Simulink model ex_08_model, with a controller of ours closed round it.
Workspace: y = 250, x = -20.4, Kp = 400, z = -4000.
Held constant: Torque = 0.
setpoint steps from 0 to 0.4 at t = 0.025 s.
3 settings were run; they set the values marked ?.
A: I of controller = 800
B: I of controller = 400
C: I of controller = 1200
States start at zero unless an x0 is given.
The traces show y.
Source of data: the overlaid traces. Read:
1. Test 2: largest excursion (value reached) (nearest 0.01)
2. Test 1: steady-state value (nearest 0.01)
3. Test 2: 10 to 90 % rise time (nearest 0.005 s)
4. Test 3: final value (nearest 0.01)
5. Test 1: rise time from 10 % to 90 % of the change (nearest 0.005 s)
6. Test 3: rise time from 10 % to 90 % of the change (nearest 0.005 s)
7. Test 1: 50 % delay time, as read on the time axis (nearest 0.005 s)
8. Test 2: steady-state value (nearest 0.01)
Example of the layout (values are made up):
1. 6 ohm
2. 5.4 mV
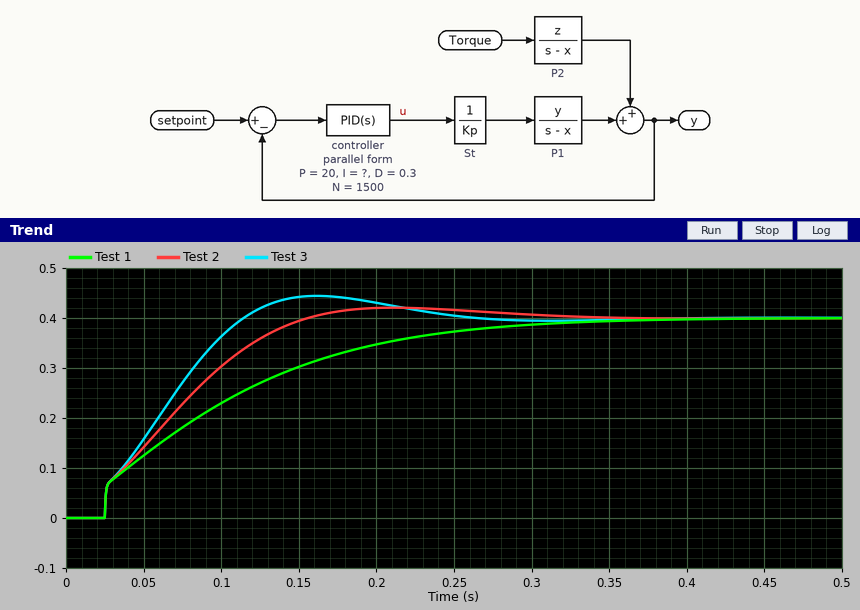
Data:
1. 0.42
2. 0.40
3. 0.100 s
4. 0.40
5. 0.195 s
6. 0.075 s
7. 0.085 s
8. 0.40
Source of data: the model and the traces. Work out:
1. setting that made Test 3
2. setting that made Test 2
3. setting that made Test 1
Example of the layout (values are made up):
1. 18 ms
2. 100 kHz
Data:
1. C
2. A
3. B
